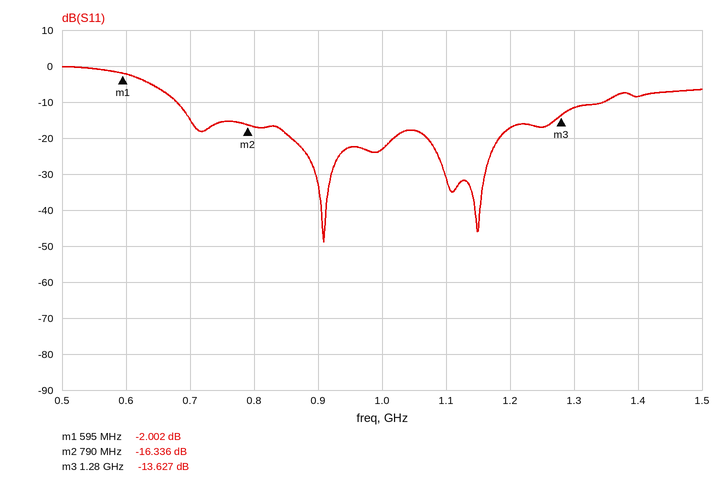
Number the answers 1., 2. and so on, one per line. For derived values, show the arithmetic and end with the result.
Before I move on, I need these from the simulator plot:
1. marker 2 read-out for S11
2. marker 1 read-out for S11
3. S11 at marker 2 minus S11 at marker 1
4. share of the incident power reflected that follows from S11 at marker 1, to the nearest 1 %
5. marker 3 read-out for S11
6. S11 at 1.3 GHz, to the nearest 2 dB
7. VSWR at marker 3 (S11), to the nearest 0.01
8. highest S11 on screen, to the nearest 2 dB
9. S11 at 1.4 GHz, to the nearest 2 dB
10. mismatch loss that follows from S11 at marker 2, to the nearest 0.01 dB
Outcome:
1. -16.336 dB
2. -2.002 dB
3. -16.336 − (-2.002) = -14.334 dB
4. 10^(-2.002/10) ≈ 63 %
5. -13.627 dB
6. -12 dB
7. (1 + 0.2083)/(1 − 0.2083) ≈ 1.53
8. 0 dB
9. -8 dB
10. −10 log10(1 − 10^(-16.336/10)) ≈ 0.10 dB
